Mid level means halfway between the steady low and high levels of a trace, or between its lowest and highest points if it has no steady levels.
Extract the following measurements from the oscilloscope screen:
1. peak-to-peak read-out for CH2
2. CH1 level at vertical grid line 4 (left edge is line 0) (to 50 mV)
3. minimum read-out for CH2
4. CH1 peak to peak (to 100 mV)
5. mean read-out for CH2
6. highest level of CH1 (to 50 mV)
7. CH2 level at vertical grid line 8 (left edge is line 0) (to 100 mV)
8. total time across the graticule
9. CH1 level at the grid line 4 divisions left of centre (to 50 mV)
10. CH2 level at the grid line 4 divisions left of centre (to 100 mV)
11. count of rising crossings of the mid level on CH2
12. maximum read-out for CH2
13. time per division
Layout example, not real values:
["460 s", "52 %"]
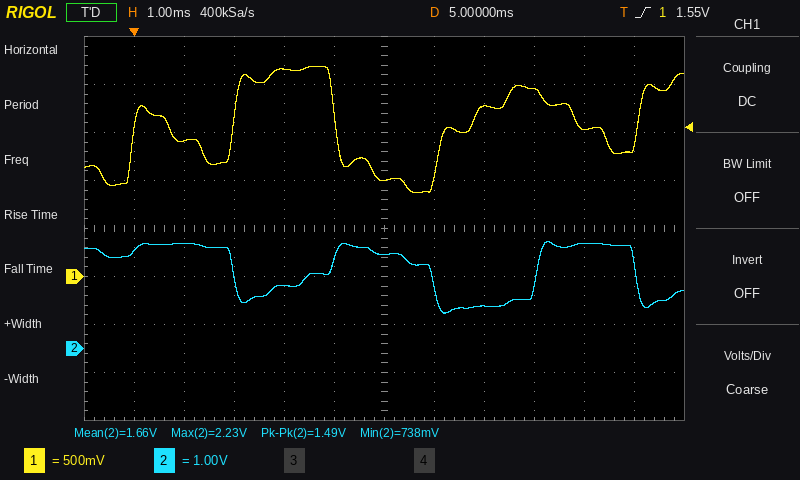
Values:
["1.49 V", "2.15 V", "738 mV", "1.30 V", "1.66 V", "2.20 V", "900 mV", "12 ms", "1.40 V", "2.2 V", "2", "2.23 V", "1 ms"]
